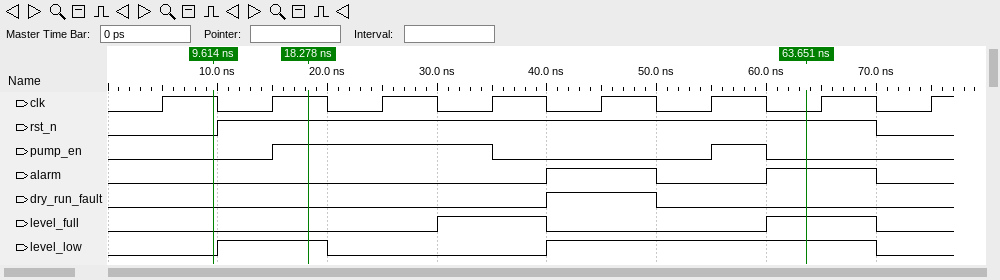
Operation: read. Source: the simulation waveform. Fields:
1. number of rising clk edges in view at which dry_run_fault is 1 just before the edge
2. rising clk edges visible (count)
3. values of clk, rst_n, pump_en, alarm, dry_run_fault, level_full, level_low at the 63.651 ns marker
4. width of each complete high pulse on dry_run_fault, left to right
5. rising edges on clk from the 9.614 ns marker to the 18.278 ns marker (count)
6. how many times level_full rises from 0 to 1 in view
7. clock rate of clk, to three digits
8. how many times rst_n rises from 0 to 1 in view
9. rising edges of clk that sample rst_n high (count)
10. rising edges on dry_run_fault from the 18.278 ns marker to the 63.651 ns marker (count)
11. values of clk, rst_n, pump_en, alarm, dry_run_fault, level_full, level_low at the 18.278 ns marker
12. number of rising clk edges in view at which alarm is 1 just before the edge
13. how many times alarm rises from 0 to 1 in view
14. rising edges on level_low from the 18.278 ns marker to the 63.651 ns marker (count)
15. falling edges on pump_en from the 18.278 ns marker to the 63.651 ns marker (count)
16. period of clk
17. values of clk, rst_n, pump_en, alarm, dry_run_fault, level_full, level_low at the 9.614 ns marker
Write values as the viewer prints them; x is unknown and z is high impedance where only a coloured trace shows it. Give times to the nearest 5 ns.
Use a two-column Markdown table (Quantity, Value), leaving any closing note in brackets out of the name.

| Quantity | Value |
|---|---|
| number of rising clk edges in view at which dry_run_fault is 1 just before the edge | 1 |
| rising clk edges visible | 8 |
| values of clk, rst_n, pump_en, alarm, dry_run_fault, level_full, level_low at the 63.651 ns marker | clk=0, rst_n=1, pump_en=0, alarm=1, dry_run_fault=0, level_full=1, level_low=1 |
| width of each complete high pulse on dry_run_fault, left to right | 10 ns |
| rising edges on clk from the 9.614 ns marker to the 18.278 ns marker | 1 |
| how many times level_full rises from 0 to 1 in view | 2 |
| clock rate of clk, to three digits | 100 MHz |
| how many times rst_n rises from 0 to 1 in view | 1 |
| rising edges of clk that sample rst_n high | 6 |
| rising edges on dry_run_fault from the 18.278 ns marker to the 63.651 ns marker | 1 |
| values of clk, rst_n, pump_en, alarm, dry_run_fault, level_full, level_low at the 18.278 ns marker | clk=1, rst_n=1, pump_en=1, alarm=0, dry_run_fault=0, level_full=0, level_low=1 |
| number of rising clk edges in view at which alarm is 1 just before the edge | 2 |
| how many times alarm rises from 0 to 1 in view | 2 |
| rising edges on level_low from the 18.278 ns marker to the 63.651 ns marker | 1 |
| falling edges on pump_en from the 18.278 ns marker to the 63.651 ns marker | 2 |
| period of clk | 10 ns |
| values of clk, rst_n, pump_en, alarm, dry_run_fault, level_full, level_low at the 9.614 ns marker | clk=1, rst_n=0, pump_en=0, alarm=0, dry_run_fault=0, level_full=0, level_low=0 |
